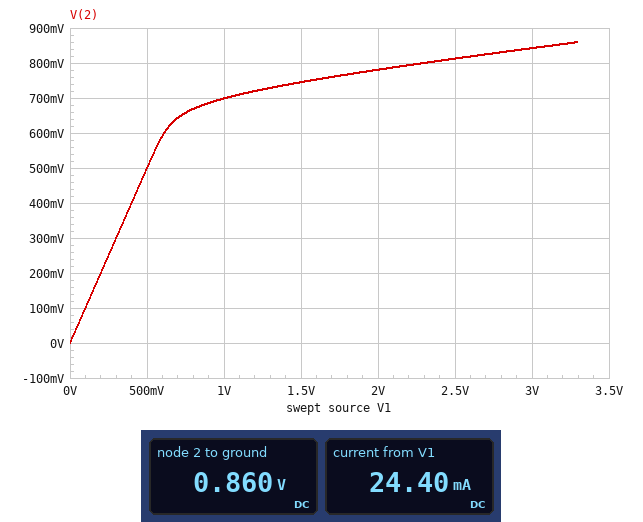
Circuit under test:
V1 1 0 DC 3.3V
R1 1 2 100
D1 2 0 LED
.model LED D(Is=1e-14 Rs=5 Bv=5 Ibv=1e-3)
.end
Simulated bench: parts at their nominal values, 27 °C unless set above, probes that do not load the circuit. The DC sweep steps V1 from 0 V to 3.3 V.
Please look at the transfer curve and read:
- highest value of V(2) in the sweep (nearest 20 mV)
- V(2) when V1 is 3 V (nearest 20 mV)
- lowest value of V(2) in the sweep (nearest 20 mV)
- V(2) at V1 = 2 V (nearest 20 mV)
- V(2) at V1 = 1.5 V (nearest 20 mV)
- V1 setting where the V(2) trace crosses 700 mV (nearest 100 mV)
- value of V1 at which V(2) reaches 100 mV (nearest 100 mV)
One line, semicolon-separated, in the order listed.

860 mV; 840 mV; 0 V; 780 mV; 740 mV; 1.0 V; 100 mV
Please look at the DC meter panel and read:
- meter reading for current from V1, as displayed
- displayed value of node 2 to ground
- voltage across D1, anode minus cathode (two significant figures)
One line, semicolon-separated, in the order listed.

24.40 mA; 0.860 V; 860 mV
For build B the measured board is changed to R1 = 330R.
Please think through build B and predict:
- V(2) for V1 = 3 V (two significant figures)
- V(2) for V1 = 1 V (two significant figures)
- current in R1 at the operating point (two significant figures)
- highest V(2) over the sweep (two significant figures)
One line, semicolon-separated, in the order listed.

740 mV; 660 mV; 7.7 mA; 750 mV
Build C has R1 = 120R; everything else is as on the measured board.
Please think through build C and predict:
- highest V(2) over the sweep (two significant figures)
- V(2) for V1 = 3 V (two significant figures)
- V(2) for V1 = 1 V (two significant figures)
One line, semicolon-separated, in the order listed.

840 mV; 820 mV; 690 mV
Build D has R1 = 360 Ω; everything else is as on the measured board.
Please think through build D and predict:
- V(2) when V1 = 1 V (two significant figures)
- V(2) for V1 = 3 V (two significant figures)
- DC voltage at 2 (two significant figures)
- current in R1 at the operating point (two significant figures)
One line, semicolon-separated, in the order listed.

660 mV; 730 mV; 740 mV; 7.1 mA
